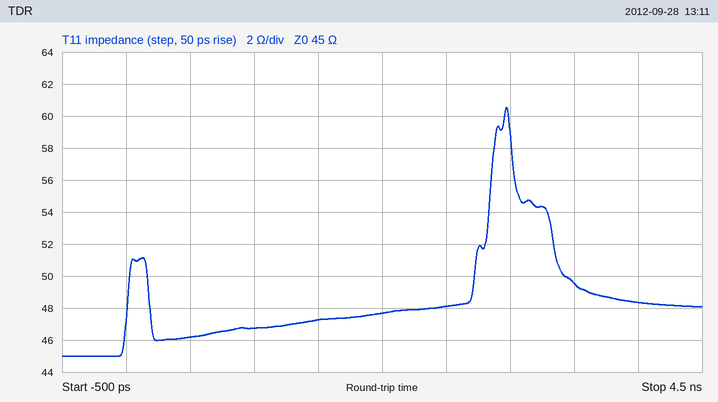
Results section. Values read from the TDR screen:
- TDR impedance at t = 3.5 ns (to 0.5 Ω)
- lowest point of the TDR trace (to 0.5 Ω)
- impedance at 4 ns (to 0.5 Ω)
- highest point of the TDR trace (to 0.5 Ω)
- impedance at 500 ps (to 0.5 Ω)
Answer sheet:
49.5 Ω
45.0 Ω
48.5 Ω
60.5 Ω
46.0 Ω
